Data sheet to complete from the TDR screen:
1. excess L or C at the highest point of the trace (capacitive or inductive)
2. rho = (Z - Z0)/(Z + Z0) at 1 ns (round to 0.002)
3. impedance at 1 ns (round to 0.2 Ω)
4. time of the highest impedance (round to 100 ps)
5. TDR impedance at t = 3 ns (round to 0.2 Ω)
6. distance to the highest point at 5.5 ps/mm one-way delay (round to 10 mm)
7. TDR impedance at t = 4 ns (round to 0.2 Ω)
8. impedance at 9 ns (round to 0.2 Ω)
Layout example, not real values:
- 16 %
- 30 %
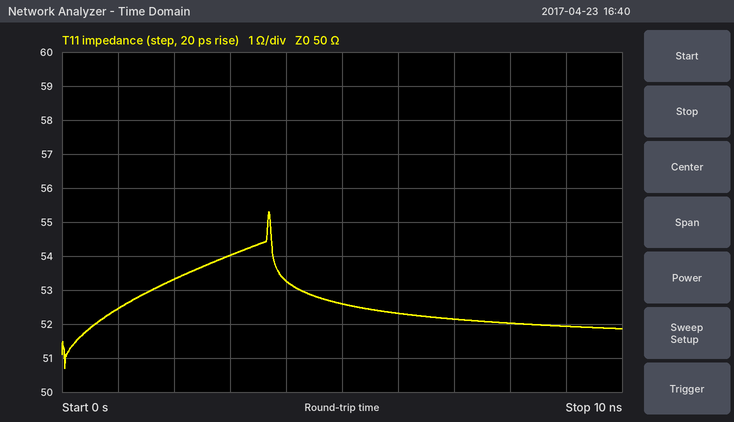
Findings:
- inductive
- +0.024
- 52.4 Ω
- 3.7 ns
- 54.0 Ω
- 340 mm
- 53.2 Ω
- 52.0 Ω
